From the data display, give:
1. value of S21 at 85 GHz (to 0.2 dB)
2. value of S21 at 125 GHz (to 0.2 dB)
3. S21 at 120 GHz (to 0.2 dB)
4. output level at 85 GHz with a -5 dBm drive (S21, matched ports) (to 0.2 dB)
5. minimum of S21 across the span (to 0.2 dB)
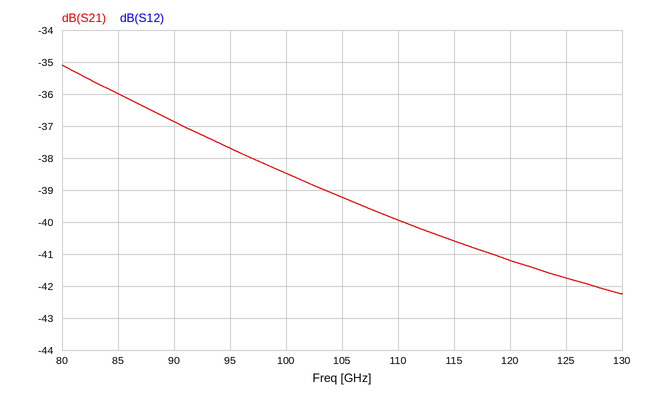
-36.0 dB
-41.8 dB
-41.2 dB
-41.0 dBm
-42.2 dB
